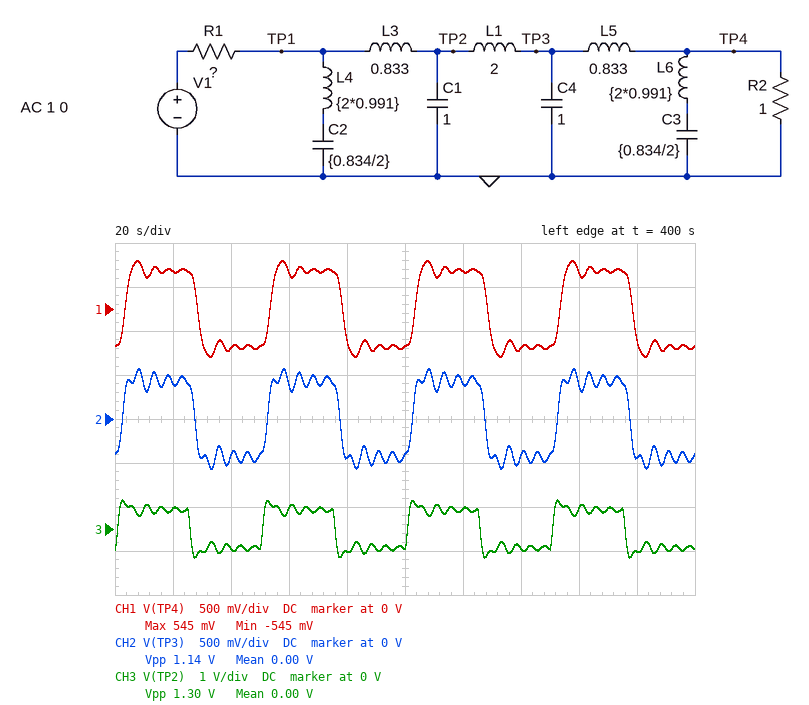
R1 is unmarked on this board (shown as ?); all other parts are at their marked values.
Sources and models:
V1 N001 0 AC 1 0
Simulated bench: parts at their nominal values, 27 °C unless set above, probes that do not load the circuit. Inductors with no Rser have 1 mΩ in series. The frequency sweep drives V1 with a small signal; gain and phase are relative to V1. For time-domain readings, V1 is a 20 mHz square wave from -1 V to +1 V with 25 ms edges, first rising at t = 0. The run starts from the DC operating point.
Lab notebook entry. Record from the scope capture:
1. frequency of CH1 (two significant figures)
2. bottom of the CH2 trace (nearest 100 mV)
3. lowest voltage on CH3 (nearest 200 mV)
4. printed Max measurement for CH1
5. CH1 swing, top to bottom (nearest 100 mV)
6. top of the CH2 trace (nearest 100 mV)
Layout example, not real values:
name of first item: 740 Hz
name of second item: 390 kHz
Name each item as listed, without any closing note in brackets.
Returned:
frequency of CH1: 20 mHz
bottom of the CH2 trace: -600 mV
lowest voltage on CH3: -600 mV
printed Max measurement for CH1: 545 mV
CH1 swing, top to bottom: 1.1 V
top of the CH2 trace: 600 mV
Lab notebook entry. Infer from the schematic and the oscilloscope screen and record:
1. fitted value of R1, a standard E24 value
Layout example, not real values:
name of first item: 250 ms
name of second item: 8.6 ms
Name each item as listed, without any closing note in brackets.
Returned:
fitted value of R1, a standard E24 value: 1.3 Ω
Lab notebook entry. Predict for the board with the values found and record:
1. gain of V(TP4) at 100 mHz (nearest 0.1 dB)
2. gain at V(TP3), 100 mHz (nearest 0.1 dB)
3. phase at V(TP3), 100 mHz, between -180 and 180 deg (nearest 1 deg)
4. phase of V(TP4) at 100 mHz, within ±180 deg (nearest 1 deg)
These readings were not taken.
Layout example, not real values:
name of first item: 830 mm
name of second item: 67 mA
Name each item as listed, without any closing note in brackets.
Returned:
gain of V(TP4) at 100 mHz: -7.6 dB
gain at V(TP3), 100 mHz: -8.0 dB
phase at V(TP3), 100 mHz, between -180 and 180 deg: -97 deg
phase of V(TP4) at 100 mHz, within ±180 deg: -131 deg
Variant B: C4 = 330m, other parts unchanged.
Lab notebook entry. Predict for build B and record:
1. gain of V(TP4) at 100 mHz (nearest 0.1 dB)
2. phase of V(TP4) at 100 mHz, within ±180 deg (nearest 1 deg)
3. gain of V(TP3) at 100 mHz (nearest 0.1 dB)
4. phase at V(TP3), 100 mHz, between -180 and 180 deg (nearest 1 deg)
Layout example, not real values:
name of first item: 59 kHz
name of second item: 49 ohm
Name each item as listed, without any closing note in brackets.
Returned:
gain of V(TP4) at 100 mHz: -8.2 dB
phase of V(TP4) at 100 mHz, within ±180 deg: -118 deg
gain of V(TP3) at 100 mHz: -8.6 dB
phase at V(TP3), 100 mHz, between -180 and 180 deg: -85 deg
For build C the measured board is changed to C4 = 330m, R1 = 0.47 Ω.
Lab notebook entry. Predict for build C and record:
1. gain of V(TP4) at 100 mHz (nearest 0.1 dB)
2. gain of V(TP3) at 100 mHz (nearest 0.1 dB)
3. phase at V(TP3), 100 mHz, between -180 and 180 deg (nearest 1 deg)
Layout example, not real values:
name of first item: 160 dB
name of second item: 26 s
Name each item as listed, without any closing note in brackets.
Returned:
gain of V(TP4) at 100 mHz: -5.6 dB
gain of V(TP3) at 100 mHz: -6.0 dB
phase at V(TP3), 100 mHz, between -180 and 180 deg: -74 deg
